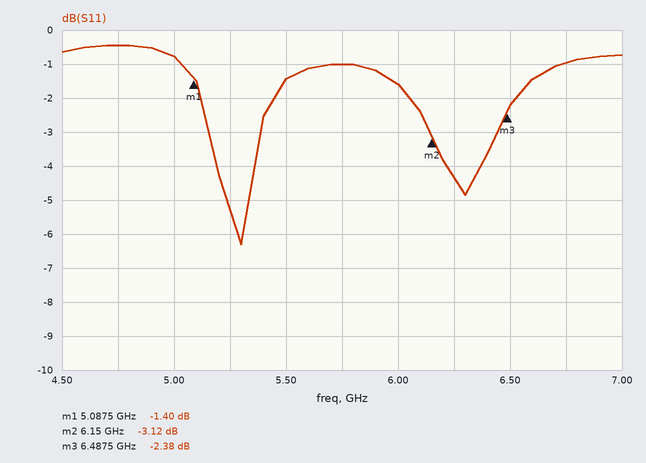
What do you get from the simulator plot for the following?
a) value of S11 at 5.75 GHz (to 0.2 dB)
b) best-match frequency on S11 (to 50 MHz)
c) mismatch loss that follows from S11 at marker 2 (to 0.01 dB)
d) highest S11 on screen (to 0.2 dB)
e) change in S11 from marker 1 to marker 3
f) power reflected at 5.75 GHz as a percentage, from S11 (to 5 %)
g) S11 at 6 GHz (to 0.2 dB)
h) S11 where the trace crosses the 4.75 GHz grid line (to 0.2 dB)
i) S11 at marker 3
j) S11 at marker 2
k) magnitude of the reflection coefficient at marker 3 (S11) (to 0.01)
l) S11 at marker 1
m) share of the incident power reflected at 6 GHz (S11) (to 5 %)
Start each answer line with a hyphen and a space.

- -1.0 dB
- 5.30 GHz
- 2.90 dB
- -0.4 dB
- -0.98 dB
- 80 %
- -1.6 dB
- -0.4 dB
- -2.38 dB
- -3.12 dB
- 0.76
- -1.40 dB
- 70 %
